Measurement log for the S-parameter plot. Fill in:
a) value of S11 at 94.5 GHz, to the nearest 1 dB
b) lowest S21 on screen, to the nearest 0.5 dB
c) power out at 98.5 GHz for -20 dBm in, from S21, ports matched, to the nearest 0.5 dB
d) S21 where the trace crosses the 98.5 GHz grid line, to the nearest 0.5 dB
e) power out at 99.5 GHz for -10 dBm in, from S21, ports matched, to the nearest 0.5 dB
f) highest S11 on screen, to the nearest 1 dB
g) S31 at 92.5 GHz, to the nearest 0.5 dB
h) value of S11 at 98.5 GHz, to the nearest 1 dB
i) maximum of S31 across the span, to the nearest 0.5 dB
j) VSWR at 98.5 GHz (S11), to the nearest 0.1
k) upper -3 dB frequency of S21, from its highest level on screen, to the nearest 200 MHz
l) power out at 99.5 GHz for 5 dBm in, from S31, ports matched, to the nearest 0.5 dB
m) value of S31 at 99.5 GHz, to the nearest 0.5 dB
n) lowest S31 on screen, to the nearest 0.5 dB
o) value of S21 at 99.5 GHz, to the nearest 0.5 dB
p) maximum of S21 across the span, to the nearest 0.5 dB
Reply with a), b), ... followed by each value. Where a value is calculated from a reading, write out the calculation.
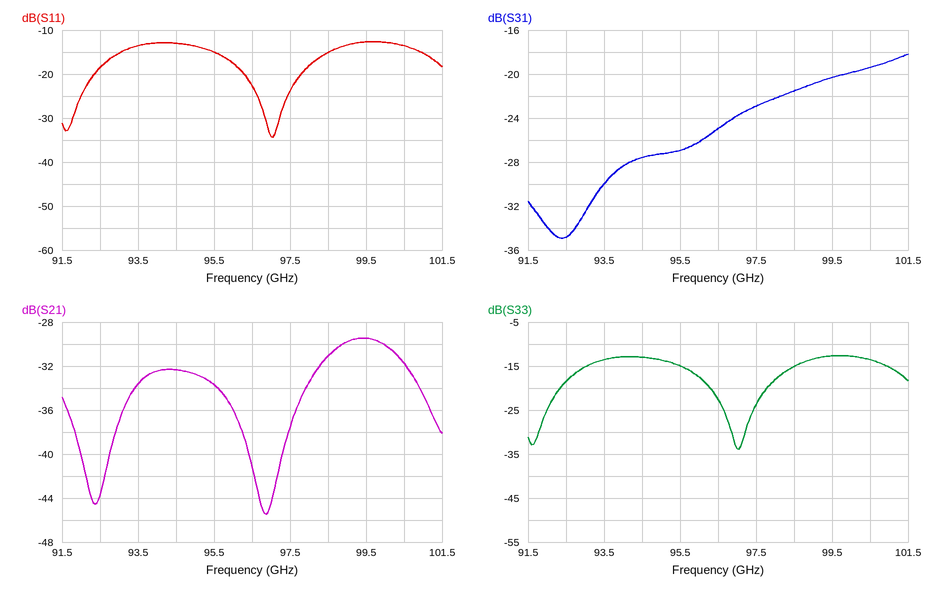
a) -13 dB
b) -45.5 dB
c) -20 dBm + (-31.0 dB) = -51.0 dBm
d) -31.0 dB
e) -10 dBm + (-29.5 dB) = -39.5 dBm
f) -13 dB
g) -35.0 dB
h) -15 dB
i) -18.0 dB
j) |Γ| = 10^(-15/20) = 0.1778; VSWR = (1 + 0.1778)/(1 − 0.1778) ≈ 1.4
k) 100.6 GHz
l) 5 dBm + (-20.5 dB) = -15.5 dBm
m) -20.5 dB
n) -35.0 dB
o) -29.5 dB
p) -29.5 dB
